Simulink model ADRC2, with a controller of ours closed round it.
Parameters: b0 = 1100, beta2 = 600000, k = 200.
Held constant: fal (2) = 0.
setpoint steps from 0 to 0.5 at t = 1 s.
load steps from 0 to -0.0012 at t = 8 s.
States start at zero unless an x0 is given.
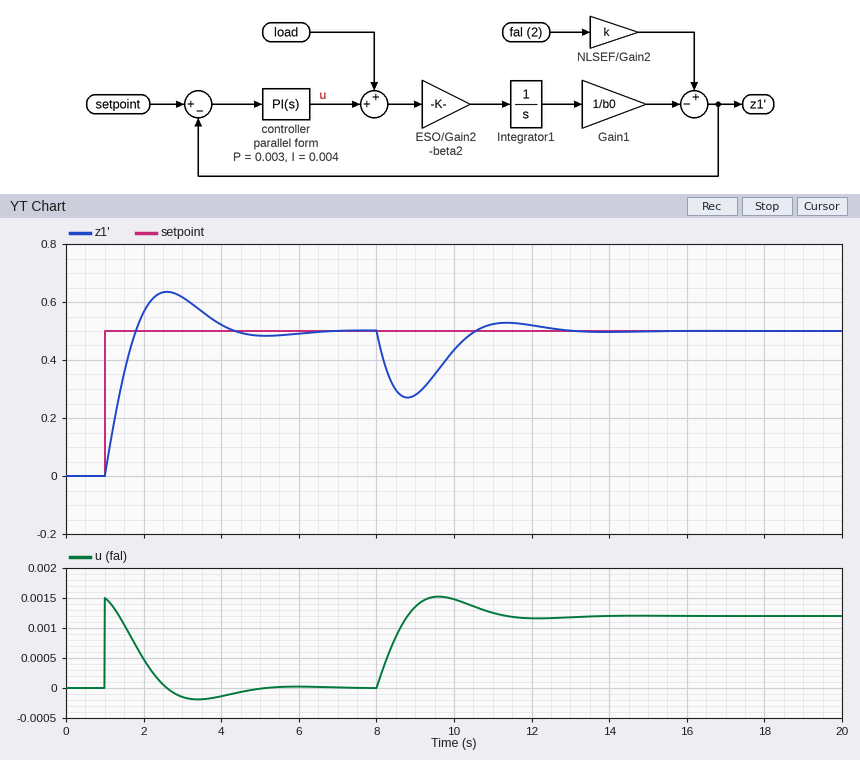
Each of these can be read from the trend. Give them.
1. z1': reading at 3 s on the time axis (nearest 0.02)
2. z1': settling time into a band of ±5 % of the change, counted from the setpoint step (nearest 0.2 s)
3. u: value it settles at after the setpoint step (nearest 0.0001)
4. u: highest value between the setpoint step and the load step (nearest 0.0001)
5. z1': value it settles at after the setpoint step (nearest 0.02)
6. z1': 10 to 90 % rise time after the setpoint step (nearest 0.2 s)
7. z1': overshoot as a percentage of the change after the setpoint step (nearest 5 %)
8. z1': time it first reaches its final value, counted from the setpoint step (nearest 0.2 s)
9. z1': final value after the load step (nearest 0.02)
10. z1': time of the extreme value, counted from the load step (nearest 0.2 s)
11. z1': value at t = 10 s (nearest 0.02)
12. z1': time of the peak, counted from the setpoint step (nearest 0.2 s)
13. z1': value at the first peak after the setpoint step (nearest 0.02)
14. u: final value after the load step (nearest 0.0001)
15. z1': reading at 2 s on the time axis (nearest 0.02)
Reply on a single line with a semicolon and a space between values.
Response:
0.62; 3.0 s; 0.0000; 0.0015; 0.50; 0.6 s; 25 %; 0.8 s; 0.50; 0.8 s; 0.44; 1.6 s; 0.64; 0.0012; 0.56
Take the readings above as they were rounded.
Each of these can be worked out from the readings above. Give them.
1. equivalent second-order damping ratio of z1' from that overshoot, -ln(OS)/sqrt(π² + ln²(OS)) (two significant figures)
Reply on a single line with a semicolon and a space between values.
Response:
0.40
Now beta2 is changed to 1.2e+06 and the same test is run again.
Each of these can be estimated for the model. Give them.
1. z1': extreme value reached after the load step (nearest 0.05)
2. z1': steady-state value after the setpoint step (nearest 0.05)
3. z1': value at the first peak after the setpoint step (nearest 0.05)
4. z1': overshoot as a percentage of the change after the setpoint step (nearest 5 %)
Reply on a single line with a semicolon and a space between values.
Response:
0.25; 0.50; 0.60; 20 %
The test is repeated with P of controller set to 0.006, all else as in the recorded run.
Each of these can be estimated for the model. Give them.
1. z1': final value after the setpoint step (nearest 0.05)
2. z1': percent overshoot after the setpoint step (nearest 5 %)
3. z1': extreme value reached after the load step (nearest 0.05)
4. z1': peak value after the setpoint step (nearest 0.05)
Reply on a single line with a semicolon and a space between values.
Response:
0.50; 10 %; 0.35; 0.55
